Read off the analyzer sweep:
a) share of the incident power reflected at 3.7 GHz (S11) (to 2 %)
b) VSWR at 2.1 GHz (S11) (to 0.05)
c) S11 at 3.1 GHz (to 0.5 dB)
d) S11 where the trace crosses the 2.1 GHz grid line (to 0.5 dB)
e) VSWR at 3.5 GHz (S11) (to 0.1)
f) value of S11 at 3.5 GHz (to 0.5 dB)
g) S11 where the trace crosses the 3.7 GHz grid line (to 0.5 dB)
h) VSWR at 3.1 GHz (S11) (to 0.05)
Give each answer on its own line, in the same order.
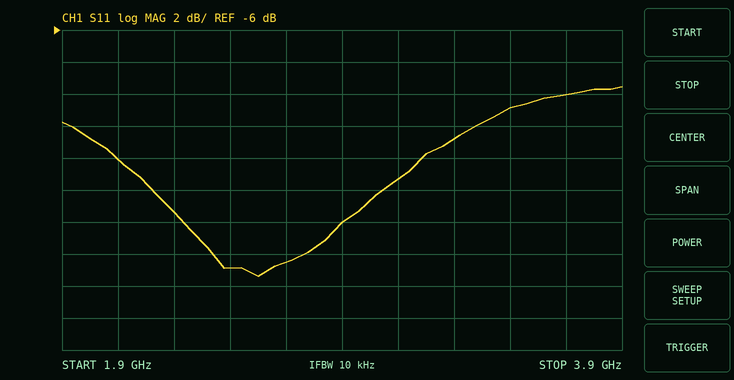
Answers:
10 %
1.50
-15.5 dB
-14.0 dB
1.8
-11.0 dB
-10.0 dB
1.40
